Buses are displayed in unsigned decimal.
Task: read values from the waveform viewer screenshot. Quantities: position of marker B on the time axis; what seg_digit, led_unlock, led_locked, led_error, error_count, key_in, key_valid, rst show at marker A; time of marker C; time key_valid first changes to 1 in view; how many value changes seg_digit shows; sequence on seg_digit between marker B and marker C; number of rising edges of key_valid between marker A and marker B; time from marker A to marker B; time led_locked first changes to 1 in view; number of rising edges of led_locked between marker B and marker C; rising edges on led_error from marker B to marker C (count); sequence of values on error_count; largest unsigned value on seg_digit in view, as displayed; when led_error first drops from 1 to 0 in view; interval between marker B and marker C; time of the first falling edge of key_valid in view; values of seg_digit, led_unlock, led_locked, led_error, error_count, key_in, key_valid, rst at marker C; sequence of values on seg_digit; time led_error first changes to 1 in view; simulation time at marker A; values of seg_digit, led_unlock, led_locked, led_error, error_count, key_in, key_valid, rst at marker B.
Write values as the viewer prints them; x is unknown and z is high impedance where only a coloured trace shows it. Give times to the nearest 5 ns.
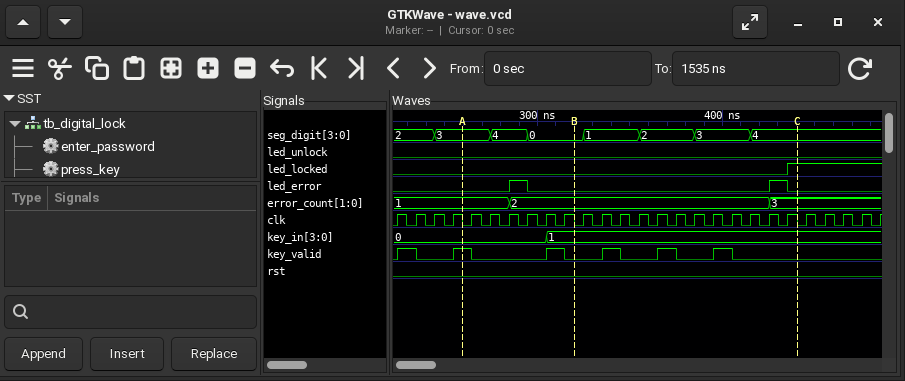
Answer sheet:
320 ns
seg_digit=3, led_unlock=0, led_locked=0, led_error=0, error_count=1, key_in=0, key_valid=1, rst=0
440 ns
225 ns
7
0, 1, 2, 3, 4
1
60 ns
435 ns
1
1
1, 2, 3
4
295 ns
120 ns
235 ns
seg_digit=4, led_unlock=0, led_locked=1, led_error=0, error_count=3, key_in=1, key_valid=0, rst=0
2, 3, 4, 0, 1, 2, 3, 4
285 ns
260 ns
seg_digit=0, led_unlock=0, led_locked=0, led_error=0, error_count=2, key_in=1, key_valid=0, rst=0
